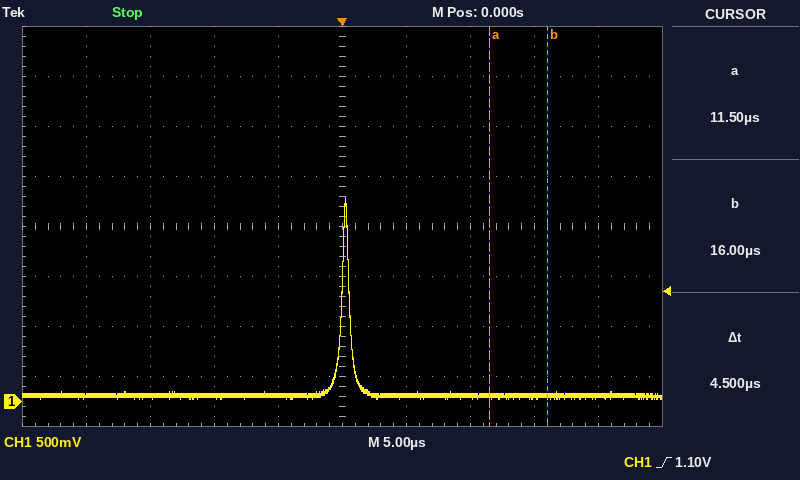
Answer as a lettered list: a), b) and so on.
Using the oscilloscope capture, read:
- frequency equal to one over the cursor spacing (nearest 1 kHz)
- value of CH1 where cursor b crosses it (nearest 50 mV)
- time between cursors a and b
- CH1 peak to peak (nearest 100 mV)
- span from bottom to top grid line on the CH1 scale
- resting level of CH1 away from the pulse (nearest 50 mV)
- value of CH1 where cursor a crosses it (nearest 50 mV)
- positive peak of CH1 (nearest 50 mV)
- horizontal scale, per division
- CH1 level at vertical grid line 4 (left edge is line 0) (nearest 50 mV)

a) 222 kHz
b) 50 mV
c) 4.5 µs
d) 2.00 V
e) 4 V
f) 50 mV
g) 50 mV
h) 2.05 V
i) 5 µs
j) 50 mV
